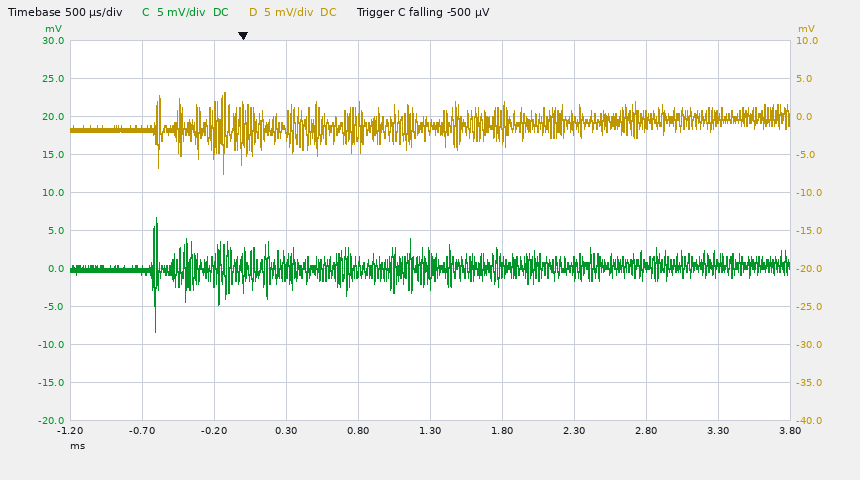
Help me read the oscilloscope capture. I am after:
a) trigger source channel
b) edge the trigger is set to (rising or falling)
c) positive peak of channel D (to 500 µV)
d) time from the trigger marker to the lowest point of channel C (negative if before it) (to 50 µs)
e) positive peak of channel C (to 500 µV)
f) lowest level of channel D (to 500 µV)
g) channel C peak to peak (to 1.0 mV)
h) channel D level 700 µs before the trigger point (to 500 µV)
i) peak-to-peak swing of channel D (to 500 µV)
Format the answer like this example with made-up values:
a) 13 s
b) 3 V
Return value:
a) channel C
b) falling
c) 3.0 mV
d) -600 µs
e) 6.5 mV
f) -7.5 mV
g) 15.0 mV
h) -1.5 mV
i) 10.5 mV
